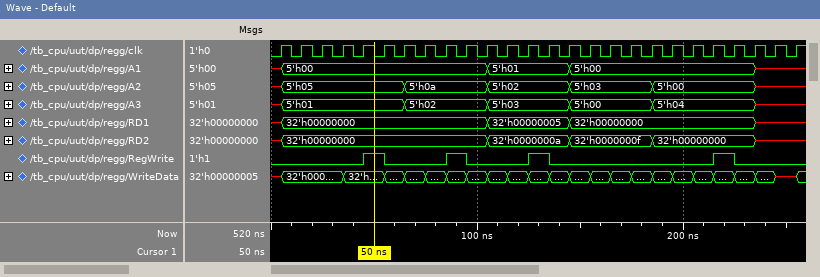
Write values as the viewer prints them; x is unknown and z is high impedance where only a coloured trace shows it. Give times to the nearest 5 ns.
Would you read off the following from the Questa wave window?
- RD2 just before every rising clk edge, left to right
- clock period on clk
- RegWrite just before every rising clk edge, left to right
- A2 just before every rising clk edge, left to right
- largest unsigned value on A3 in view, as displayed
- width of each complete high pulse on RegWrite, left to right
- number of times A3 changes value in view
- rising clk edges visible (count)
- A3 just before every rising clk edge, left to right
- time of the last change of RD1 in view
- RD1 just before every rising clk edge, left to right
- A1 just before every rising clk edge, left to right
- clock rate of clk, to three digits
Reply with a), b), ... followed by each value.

a) x, 32'h00000000, 32'h00000000, 32'h00000000, 32'h00000000, 32'h00000000, 32'h00000000, 32'h00000000, 32'h00000000, 32'h00000000, 32'h00000000, 32'h0000000a, 32'h0000000a, 32'h0000000a, 32'h0000000a, 32'h0000000f, 32'h0000000f, 32'h0000000f, 32'h0000000f, 32'h00000000, 32'h00000000, 32'h00000000, 32'h00000000, 32'h00000000, x, x
b) 10 ns
c) 0 0 0 0 0 1 0 0 0 1 0 0 0 1 0 0 0 0 0 0 0 0 1 0 0 0
d) x, 5'h05, 5'h05, 5'h05, 5'h05, 5'h05, 5'h05, 5'h0a, 5'h0a, 5'h0a, 5'h0a, 5'h02, 5'h02, 5'h02, 5'h02, 5'h03, 5'h03, 5'h03, 5'h03, 5'h00, 5'h00, 5'h00, 5'h00, 5'h00, x, x
e) 5'h04
f) 10 ns, 10 ns, 10 ns, 10 ns
g) 6
h) 26
i) x, 5'h01, 5'h01, 5'h01, 5'h01, 5'h01, 5'h01, 5'h02, 5'h02, 5'h02, 5'h02, 5'h03, 5'h03, 5'h03, 5'h03, 5'h00, 5'h00, 5'h00, 5'h00, 5'h04, 5'h04, 5'h04, 5'h04, 5'h04, x, x
j) 235 ns
k) x, 32'h00000000, 32'h00000000, 32'h00000000, 32'h00000000, 32'h00000000, 32'h00000000, 32'h00000000, 32'h00000000, 32'h00000000, 32'h00000000, 32'h00000005, 32'h00000005, 32'h00000005, 32'h00000005, 32'h00000000, 32'h00000000, 32'h00000000, 32'h00000000, 32'h00000000, 32'h00000000, 32'h00000000, 32'h00000000, 32'h00000000, x, x
l) x, 5'h00, 5'h00, 5'h00, 5'h00, 5'h00, 5'h00, 5'h00, 5'h00, 5'h00, 5'h00, 5'h01, 5'h01, 5'h01, 5'h01, 5'h00, 5'h00, 5'h00, 5'h00, 5'h00, 5'h00, 5'h00, 5'h00, 5'h00, x, x
m) 100 MHz
